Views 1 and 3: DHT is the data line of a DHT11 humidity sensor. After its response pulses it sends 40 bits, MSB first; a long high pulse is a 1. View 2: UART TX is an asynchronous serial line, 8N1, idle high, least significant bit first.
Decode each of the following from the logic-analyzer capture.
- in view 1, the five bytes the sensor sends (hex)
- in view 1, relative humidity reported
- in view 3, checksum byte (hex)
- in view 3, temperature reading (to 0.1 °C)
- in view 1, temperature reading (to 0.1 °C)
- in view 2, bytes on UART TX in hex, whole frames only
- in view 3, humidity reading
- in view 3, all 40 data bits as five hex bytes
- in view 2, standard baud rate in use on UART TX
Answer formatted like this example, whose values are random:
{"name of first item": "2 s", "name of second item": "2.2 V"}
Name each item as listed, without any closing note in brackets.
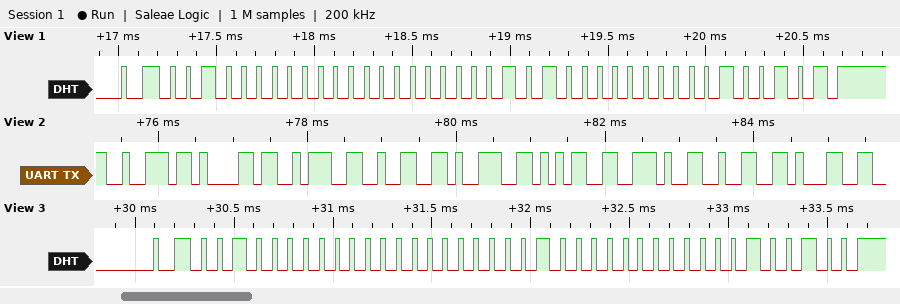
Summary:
{"in view 1, the five bytes the sensor sends": "20 00 05 00 25", "in view 1, relative humidity reported": "32 %", "in view 3, checksum byte": "0x24", "in view 3, temperature reading": "4.0 °C", "in view 1, temperature reading": "5.0 °C", "in view 2, bytes on UART TX in hex, whole frames only": "72 61 3A 32 39 35 2E 32 31", "in view 3, humidity reading": "32 %", "in view 3, all 40 data bits as five hex bytes": "20 00 04 00 24", "in view 2, standard baud rate in use on UART TX": "9600 baud"}
